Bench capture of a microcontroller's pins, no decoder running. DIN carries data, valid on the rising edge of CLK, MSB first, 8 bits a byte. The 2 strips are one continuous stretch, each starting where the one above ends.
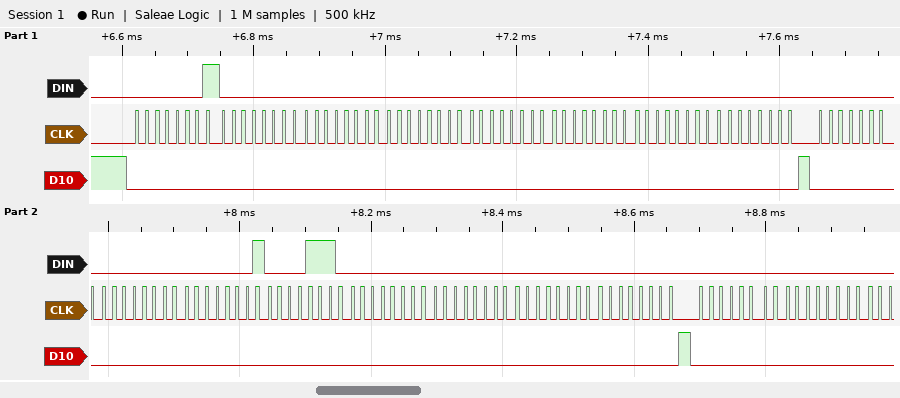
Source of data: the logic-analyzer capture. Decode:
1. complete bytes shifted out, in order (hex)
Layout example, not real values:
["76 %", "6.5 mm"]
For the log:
["0x01 0x00 0x00 0x00 0x00 0x00 0x00 0x00 0x00 0x00 0x01 0x0E 0x00 0x00 0x00 0x00 0x00 0x00"]
